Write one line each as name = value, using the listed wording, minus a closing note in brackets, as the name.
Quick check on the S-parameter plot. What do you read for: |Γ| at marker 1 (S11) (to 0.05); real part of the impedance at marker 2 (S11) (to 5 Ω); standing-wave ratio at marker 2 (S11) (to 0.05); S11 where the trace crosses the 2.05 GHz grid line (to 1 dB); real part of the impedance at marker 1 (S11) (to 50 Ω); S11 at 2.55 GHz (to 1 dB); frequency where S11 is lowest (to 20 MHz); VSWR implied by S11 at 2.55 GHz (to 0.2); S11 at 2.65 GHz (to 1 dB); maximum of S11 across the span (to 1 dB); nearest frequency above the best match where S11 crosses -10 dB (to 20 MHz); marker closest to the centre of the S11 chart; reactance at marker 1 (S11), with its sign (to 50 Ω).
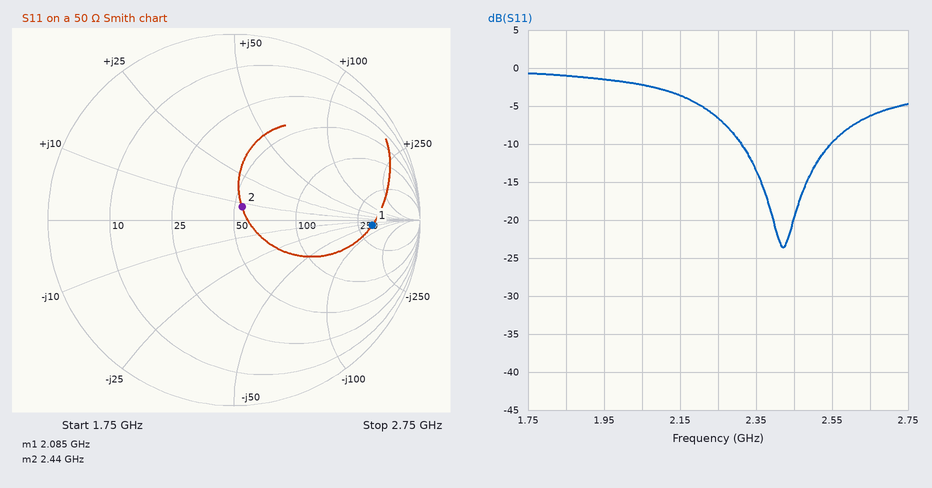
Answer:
|Γ| at marker 1 (S11) = 0.75
real part of the impedance at marker 2 (S11) = 55 Ω
standing-wave ratio at marker 2 (S11) = 1.20
S11 where the trace crosses the 2.05 GHz grid line = -2 dB
real part of the impedance at marker 1 (S11) = 350 Ω
S11 at 2.55 GHz = -10 dB
frequency where S11 is lowest = 2.42 GHz
VSWR implied by S11 at 2.55 GHz = 2.0
S11 at 2.65 GHz = -6 dB
maximum of S11 across the span = -1 dB
nearest frequency above the best match where S11 crosses -10 dB = 2.54 GHz
marker closest to the centre of the S11 chart = marker 2
reactance at marker 1 (S11), with its sign = -50 Ω
